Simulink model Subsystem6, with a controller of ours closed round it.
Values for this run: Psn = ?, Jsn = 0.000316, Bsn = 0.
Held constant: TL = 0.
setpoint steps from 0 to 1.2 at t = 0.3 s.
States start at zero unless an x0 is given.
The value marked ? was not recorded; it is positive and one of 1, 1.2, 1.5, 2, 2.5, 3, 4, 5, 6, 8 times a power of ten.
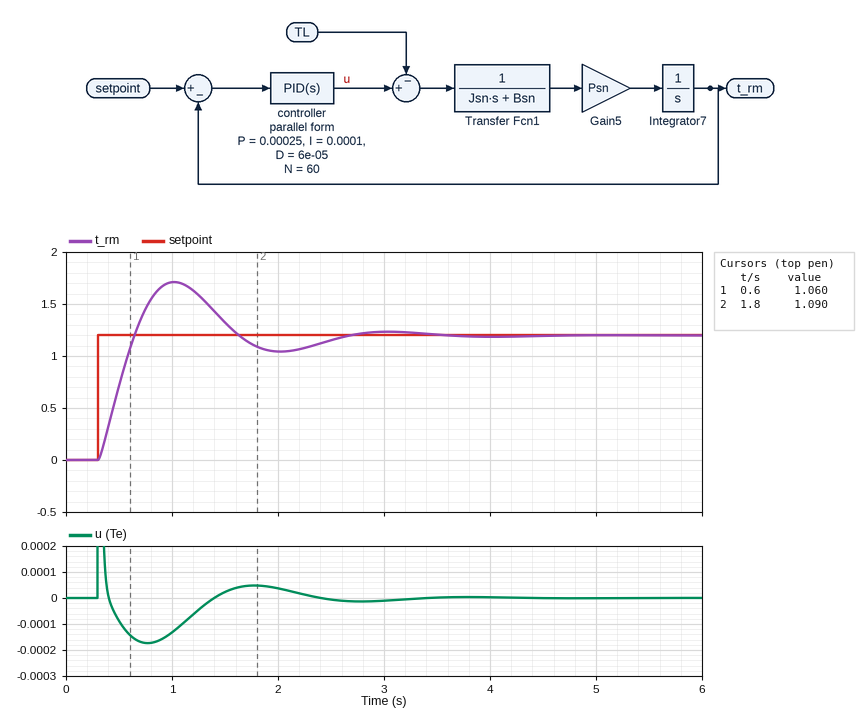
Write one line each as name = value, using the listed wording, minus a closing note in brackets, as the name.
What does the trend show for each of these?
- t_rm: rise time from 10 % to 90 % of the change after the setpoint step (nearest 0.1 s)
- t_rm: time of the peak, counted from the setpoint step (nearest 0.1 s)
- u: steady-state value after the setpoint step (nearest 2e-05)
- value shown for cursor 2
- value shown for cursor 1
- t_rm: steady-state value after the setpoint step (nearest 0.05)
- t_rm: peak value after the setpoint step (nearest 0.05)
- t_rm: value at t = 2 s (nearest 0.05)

t_rm: rise time from 10 % to 90 % of the change after the setpoint step = 0.3 s
t_rm: time of the peak, counted from the setpoint step = 0.7 s
u: steady-state value after the setpoint step = 0.00000
value shown for cursor 2 = 1.090
value shown for cursor 1 = 1.060
t_rm: steady-state value after the setpoint step = 1.20
t_rm: peak value after the setpoint step = 1.70
t_rm: value at t = 2 s = 1.05
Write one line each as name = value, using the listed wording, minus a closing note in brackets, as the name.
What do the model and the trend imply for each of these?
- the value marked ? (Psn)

the value marked ? = 15
